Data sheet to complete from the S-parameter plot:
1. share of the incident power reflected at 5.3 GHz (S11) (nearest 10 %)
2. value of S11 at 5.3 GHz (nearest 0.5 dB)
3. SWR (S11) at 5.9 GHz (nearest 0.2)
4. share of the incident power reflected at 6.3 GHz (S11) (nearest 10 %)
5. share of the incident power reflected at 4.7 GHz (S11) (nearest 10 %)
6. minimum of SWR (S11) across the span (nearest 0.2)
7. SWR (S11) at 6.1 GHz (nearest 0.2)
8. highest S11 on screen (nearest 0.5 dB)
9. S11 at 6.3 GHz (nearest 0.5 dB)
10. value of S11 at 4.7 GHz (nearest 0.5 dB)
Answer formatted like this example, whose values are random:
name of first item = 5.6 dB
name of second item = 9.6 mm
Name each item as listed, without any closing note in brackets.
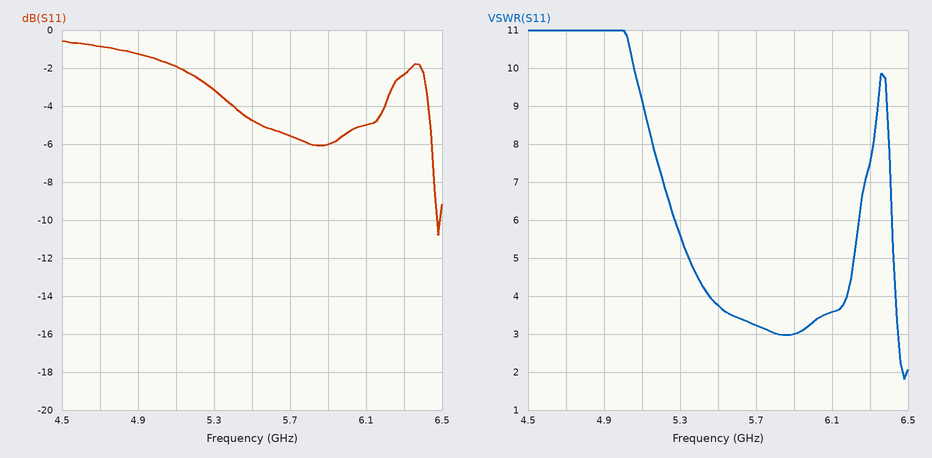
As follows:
share of the incident power reflected at 5.3 GHz (S11) = 50 %
value of S11 at 5.3 GHz = -3.0 dB
SWR (S11) at 5.9 GHz = 3.0
share of the incident power reflected at 6.3 GHz (S11) = 60 %
share of the incident power reflected at 4.7 GHz (S11) = 80 %
minimum of SWR (S11) across the span = 1.8
SWR (S11) at 6.1 GHz = 3.6
highest S11 on screen = -0.5 dB
S11 at 6.3 GHz = -2.5 dB
value of S11 at 4.7 GHz = -1.0 dB
